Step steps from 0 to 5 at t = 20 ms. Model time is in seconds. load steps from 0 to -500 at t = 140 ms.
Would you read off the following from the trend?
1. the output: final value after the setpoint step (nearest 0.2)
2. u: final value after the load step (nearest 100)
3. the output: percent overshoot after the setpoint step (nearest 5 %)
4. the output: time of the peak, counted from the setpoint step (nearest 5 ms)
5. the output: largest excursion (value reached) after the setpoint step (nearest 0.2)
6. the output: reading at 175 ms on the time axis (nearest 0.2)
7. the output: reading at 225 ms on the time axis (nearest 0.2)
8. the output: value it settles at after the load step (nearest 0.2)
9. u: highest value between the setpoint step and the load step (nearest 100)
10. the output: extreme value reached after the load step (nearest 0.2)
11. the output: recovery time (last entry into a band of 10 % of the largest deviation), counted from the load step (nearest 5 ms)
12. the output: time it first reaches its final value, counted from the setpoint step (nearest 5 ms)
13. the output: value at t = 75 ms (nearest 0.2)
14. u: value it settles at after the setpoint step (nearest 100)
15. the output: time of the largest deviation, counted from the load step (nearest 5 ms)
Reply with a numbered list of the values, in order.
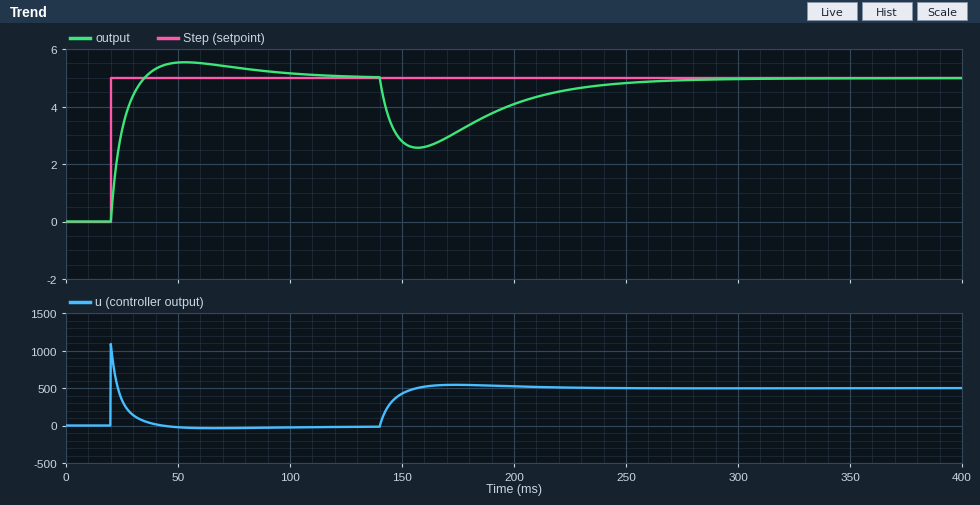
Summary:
1. 5.0
2. 500
3. 10 %
4. 35 ms
5. 5.6
6. 3.2
7. 4.6
8. 5.0
9. 1100
10. 2.6
11. 100 ms
12. 15 ms
13. 5.4
14. 0
15. 15 ms
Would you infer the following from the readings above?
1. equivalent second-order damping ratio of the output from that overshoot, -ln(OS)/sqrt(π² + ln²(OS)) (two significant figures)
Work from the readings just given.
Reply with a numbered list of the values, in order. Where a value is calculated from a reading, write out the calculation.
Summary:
1. ln(0.1) = -2.303; 2.303 / sqrt(9.870 + 5.302) = 0.59
